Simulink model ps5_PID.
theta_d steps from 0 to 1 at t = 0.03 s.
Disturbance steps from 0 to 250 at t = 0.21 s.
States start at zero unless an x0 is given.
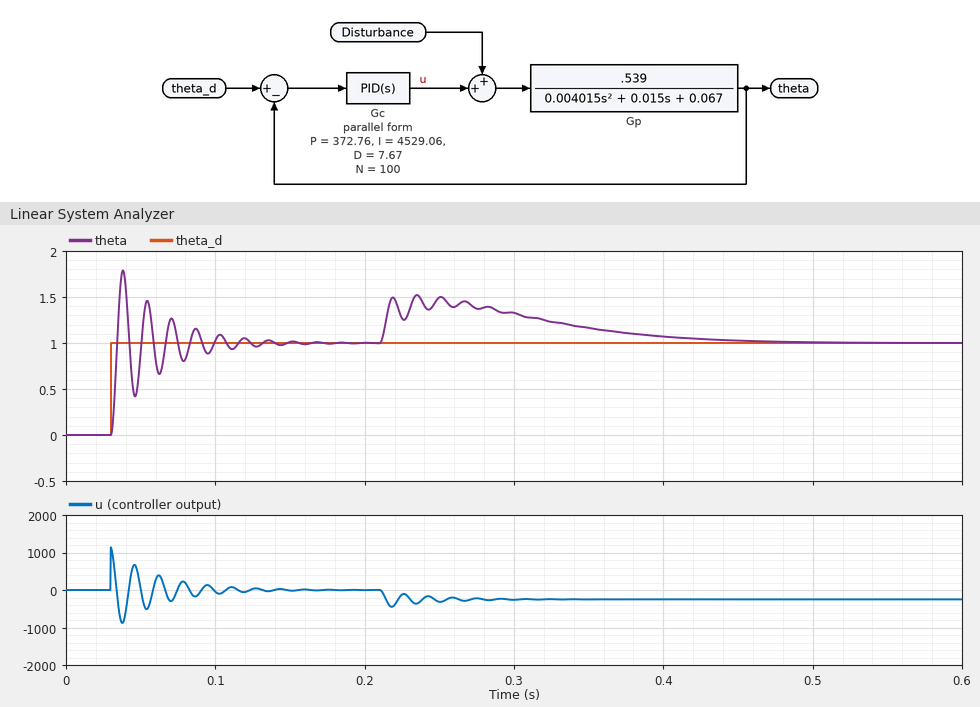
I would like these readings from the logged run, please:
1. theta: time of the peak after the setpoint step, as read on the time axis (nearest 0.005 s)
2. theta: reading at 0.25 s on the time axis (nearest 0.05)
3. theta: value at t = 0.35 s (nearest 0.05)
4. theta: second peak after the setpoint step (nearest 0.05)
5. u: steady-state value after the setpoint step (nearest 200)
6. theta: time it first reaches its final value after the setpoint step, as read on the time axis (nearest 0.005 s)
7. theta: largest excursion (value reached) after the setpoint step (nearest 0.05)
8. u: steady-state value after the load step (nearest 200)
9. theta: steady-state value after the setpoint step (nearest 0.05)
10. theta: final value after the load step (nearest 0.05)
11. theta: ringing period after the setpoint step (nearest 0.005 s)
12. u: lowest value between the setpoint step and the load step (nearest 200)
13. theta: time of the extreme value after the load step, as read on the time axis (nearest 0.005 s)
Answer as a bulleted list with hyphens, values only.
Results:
- 0.040 s
- 1.50
- 1.15
- 1.45
- 0
- 0.035 s
- 1.80
- -200
- 1.00
- 1.00
- 0.015 s
- -800
- 0.235 s
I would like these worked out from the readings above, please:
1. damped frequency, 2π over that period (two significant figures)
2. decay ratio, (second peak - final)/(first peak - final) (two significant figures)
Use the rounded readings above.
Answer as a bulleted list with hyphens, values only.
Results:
- 420 rad/s
- 0.56
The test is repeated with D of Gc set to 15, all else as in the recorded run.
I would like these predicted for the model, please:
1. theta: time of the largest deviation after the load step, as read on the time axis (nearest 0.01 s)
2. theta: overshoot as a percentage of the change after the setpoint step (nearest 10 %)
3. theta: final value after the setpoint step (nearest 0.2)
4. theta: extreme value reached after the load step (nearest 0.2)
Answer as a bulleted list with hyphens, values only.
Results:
- 0.27 s
- 80 %
- 1.0
- 1.4
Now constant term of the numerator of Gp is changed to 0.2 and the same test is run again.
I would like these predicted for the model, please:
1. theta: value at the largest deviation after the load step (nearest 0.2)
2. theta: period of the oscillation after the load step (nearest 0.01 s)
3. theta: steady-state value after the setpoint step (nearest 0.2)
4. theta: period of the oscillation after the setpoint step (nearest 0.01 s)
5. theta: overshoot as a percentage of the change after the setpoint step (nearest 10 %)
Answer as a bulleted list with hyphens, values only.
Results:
- 1.6
- 0.03 s
- 1.0
- 0.03 s
- 70 %
